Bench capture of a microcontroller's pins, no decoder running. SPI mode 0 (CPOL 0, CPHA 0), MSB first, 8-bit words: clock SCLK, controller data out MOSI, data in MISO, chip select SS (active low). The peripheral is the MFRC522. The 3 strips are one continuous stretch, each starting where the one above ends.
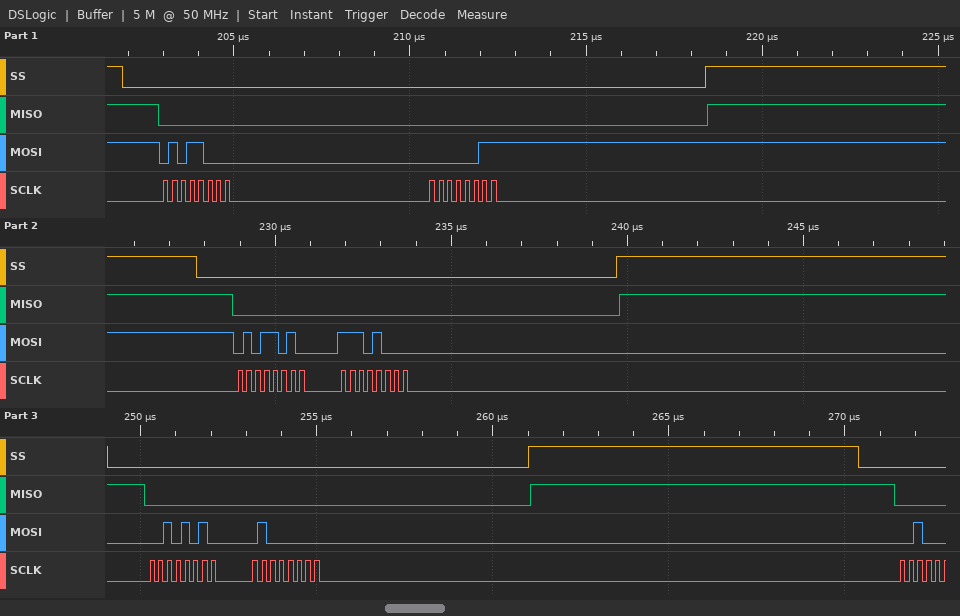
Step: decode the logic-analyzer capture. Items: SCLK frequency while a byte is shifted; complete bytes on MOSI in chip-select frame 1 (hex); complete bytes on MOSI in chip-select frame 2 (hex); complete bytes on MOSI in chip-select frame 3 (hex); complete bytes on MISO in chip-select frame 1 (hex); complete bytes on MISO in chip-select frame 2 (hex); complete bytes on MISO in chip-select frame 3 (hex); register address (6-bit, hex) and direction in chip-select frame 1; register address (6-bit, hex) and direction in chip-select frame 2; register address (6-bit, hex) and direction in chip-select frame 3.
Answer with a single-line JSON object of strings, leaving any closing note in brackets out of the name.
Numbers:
{"SCLK frequency while a byte is shifted": "4 MHz", "complete bytes on MOSI in chip-select frame 1": "58 03", "complete bytes on MOSI in chip-select frame 2": "5A E8", "complete bytes on MOSI in chip-select frame 3": "2A 40", "complete bytes on MISO in chip-select frame 1": "00 00", "complete bytes on MISO in chip-select frame 2": "00 00", "complete bytes on MISO in chip-select frame 3": "00 00", "register address (6-bit, hex) and direction in chip-select frame 1": "0x2C write", "register address (6-bit, hex) and direction in chip-select frame 2": "0x2D write", "register address (6-bit, hex) and direction in chip-select frame 3": "0x15 write"}
